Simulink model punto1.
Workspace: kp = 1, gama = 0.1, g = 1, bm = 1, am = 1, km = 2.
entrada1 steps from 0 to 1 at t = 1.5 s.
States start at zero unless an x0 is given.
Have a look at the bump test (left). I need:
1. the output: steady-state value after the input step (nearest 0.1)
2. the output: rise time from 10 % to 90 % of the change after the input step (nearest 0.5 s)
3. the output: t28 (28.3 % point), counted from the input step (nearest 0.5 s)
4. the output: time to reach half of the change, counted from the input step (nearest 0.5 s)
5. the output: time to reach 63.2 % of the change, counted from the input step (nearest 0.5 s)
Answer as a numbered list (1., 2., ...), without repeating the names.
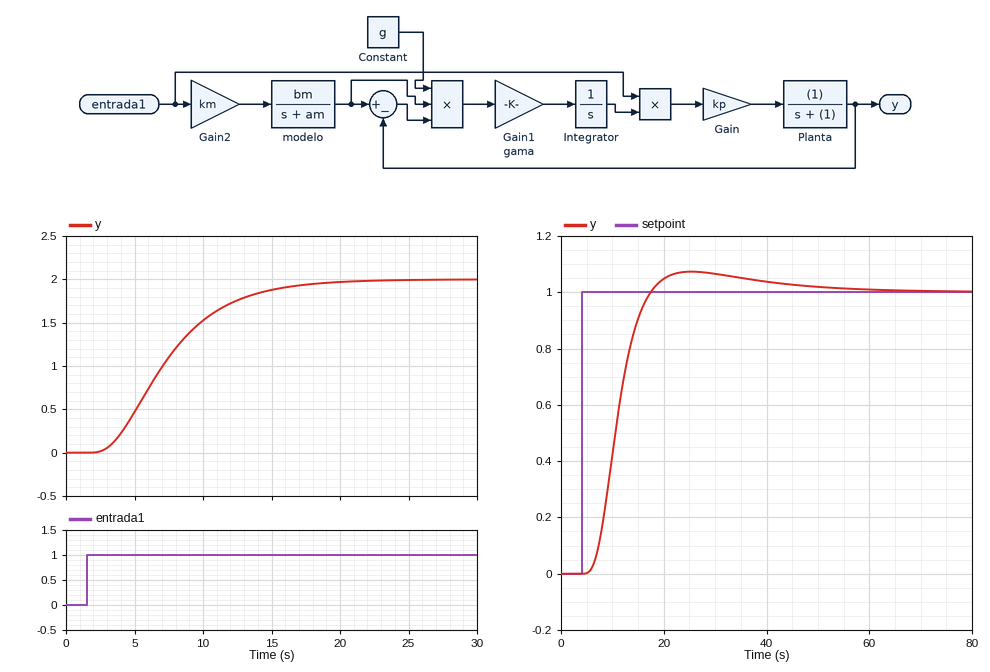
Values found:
1. 2.0
2. 9.5 s
3. 4.0 s
4. 5.5 s
5. 7.0 s
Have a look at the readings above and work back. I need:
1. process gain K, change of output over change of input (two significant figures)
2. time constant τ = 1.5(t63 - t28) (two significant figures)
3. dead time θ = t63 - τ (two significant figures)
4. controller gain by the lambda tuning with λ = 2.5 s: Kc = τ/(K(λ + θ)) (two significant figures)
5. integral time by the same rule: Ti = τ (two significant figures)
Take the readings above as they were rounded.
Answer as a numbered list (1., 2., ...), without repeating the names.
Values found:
1. 2.0
2. 4.5 s
3. 2.5 s
4. 0.45
5. 4.5 s
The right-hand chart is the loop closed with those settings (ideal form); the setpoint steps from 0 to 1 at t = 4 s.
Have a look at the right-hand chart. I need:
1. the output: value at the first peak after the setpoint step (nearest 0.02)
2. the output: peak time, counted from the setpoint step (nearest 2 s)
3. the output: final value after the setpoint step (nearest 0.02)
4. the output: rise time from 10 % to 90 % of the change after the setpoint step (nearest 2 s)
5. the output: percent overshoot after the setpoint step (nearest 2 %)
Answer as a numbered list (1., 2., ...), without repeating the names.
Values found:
1. 1.08
2. 22 s
3. 1.00
4. 8 s
5. 8 %
